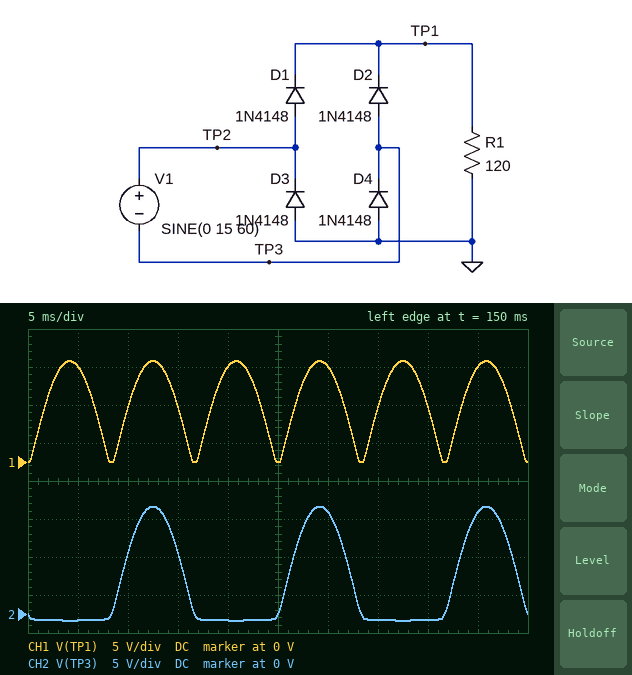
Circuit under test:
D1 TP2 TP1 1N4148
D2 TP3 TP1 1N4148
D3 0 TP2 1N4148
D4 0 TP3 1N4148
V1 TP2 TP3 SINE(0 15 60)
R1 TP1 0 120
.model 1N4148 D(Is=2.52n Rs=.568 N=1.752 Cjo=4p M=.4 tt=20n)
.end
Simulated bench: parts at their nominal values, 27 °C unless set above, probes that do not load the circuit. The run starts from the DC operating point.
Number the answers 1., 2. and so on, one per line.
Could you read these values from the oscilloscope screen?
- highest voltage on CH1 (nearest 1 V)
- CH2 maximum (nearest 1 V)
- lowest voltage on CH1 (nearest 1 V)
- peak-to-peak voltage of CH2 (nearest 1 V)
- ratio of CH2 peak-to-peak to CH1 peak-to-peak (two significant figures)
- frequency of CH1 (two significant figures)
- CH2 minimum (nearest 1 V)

1. 13 V
2. 14 V
3. 0 V
4. 15 V
5. 1.1
6. 120 Hz
7. -1 V
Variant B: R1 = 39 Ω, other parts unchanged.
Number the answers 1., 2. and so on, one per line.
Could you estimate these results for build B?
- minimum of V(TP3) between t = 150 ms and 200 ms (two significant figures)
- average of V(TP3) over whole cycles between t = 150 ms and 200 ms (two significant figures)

1. -1.0 V
2. 3.9 V
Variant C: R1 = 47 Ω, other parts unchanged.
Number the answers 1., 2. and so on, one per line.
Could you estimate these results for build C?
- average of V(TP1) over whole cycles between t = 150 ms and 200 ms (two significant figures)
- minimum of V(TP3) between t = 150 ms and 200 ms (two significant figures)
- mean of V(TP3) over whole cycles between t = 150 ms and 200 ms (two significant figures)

1. 7.8 V
2. -1.0 V
3. 3.9 V
